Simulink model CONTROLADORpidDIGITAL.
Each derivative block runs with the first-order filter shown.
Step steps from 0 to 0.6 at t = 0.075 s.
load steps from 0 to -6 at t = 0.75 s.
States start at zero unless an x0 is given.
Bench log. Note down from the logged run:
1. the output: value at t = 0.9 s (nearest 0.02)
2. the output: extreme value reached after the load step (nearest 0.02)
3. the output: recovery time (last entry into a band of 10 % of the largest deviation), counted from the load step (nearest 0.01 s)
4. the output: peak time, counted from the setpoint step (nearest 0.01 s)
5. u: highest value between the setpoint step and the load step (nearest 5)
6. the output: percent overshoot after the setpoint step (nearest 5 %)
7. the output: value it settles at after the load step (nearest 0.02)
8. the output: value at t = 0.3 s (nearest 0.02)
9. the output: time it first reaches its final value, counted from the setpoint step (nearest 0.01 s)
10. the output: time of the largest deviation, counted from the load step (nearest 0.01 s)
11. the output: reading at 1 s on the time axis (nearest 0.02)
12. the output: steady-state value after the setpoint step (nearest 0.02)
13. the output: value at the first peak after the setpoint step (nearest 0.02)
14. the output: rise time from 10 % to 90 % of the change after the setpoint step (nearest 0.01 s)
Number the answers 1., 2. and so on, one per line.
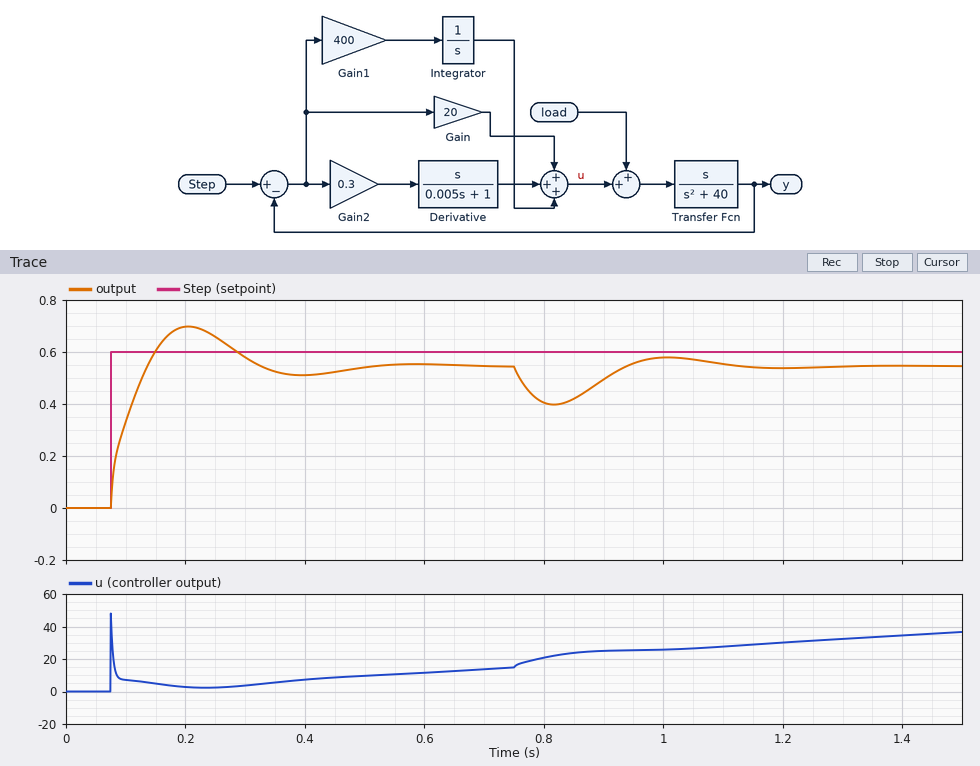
1. 0.50
2. 0.40
3. 0.33 s
4. 0.13 s
5. 50
6. 30 %
7. 0.54
8. 0.58
9. 0.06 s
10. 0.07 s
11. 0.58
12. 0.54
13. 0.70
14. 0.05 s
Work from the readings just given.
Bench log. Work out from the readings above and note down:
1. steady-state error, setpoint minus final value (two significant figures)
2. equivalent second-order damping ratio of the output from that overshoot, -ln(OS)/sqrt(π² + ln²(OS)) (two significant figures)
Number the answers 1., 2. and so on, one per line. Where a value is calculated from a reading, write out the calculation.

1. 0.6 - 0.54 = 0.060
2. ln(0.3) = -1.204; 1.204 / sqrt(9.870 + 1.450) = 0.36
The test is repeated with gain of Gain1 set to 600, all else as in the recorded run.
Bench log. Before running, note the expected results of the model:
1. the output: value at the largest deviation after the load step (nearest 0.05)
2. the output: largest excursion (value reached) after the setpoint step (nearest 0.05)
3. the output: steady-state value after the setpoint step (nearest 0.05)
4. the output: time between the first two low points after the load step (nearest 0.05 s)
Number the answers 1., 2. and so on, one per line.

1. 0.45
2. 0.75
3. 0.55
4. 0.30 s
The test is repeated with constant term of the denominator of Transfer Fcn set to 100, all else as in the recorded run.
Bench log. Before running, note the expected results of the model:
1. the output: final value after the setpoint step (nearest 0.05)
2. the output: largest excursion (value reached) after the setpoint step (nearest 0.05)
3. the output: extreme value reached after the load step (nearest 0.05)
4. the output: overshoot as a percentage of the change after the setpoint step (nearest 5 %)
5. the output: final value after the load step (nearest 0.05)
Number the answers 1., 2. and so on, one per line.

1. 0.50
2. 0.65
3. 0.35
4. 30 %
5. 0.50
